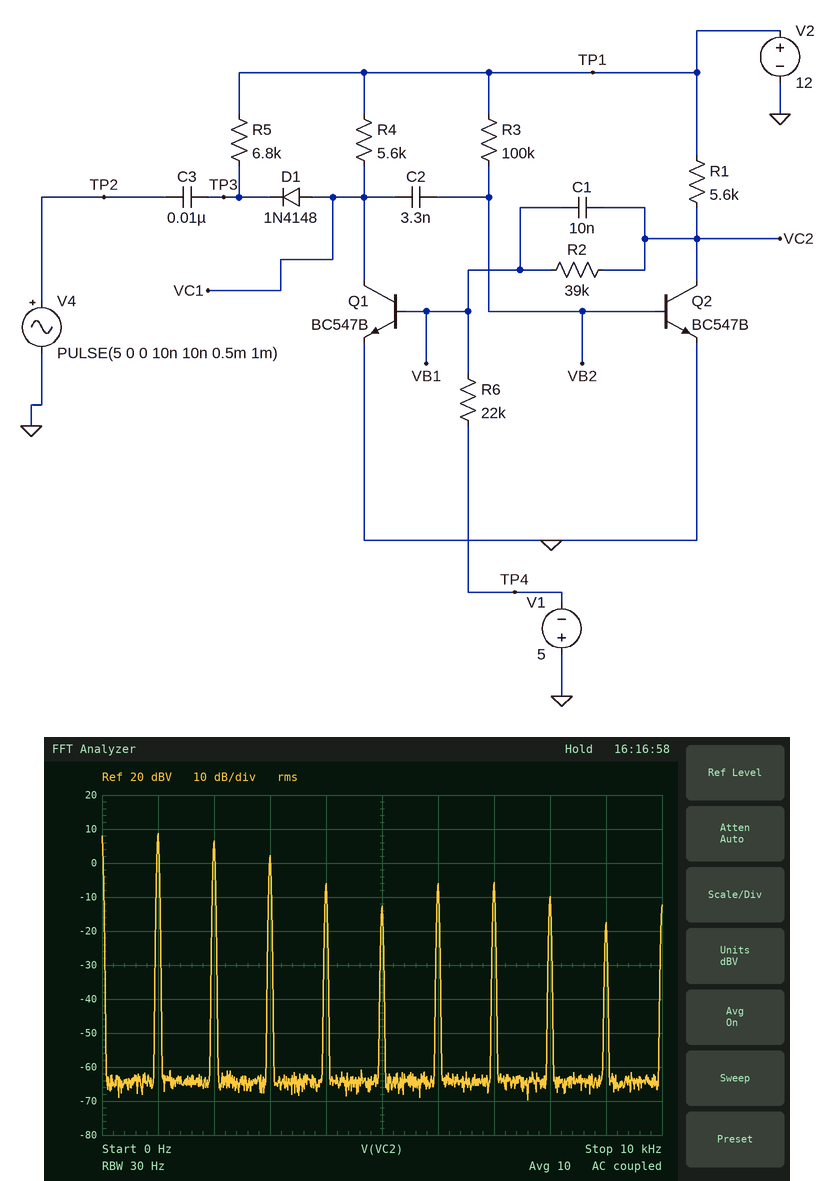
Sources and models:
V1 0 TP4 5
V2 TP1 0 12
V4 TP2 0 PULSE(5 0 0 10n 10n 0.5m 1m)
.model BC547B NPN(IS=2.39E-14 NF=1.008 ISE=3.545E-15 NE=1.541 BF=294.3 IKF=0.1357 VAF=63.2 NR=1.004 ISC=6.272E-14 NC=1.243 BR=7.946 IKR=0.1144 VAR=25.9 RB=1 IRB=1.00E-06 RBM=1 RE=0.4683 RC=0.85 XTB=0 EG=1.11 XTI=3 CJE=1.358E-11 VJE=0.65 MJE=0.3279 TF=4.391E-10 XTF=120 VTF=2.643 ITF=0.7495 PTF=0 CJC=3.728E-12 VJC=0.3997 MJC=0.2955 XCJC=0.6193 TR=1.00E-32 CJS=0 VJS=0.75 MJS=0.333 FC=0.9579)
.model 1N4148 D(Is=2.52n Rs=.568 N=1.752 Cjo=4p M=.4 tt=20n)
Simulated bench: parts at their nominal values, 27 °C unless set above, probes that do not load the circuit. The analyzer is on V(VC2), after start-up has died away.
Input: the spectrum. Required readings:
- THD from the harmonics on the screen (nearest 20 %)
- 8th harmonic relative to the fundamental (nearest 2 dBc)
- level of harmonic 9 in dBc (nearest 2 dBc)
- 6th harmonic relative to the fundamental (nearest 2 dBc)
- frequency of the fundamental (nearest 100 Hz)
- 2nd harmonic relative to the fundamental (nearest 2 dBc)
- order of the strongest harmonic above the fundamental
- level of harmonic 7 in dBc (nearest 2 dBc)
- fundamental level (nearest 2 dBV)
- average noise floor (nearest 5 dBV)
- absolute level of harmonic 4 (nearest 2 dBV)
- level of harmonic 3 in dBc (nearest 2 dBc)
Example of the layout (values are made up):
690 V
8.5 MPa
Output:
100 %
-18 dBc
-26 dBc
-14 dBc
1.0 kHz
-2 dBc
2
-14 dBc
8 dBV
-65 dBV
-6 dBV
-6 dBc
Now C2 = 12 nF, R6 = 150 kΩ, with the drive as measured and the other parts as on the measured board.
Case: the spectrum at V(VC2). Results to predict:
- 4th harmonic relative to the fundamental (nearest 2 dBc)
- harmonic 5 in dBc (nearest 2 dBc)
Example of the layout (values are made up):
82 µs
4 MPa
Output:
-12 dBc
-26 dBc
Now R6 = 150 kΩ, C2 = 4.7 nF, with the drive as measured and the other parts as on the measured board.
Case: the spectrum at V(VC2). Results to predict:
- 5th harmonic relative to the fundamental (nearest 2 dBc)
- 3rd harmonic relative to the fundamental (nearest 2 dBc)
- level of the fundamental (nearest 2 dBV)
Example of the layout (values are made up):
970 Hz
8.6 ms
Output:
-14 dBc
-20 dBc
12 dBV
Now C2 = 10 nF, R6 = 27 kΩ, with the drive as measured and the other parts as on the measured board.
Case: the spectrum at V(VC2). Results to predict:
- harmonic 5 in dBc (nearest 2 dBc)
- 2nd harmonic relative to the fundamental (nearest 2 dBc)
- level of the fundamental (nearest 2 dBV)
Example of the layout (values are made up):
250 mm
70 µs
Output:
-14 dBc
-6 dBc
12 dBV
